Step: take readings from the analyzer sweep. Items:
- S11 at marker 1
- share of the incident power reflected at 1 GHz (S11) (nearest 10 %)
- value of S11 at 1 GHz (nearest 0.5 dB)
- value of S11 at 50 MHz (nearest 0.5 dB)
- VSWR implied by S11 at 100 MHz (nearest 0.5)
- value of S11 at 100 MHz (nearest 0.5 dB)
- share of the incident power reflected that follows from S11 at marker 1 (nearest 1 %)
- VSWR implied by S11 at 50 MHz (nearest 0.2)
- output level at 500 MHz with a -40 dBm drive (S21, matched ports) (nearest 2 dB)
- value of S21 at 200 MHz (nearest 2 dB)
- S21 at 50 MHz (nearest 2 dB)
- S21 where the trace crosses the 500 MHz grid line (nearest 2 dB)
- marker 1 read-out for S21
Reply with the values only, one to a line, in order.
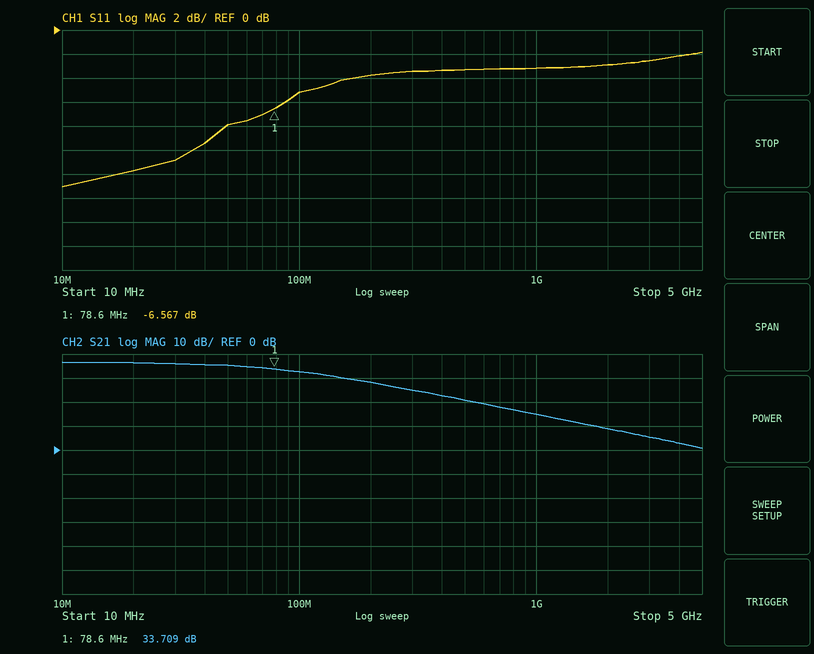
-6.567 dB
50 %
-3.0 dB
-8.0 dB
3.5
-5.0 dB
22 %
2.4
-20 dBm
28 dB
36 dB
20 dB
33.709 dB
